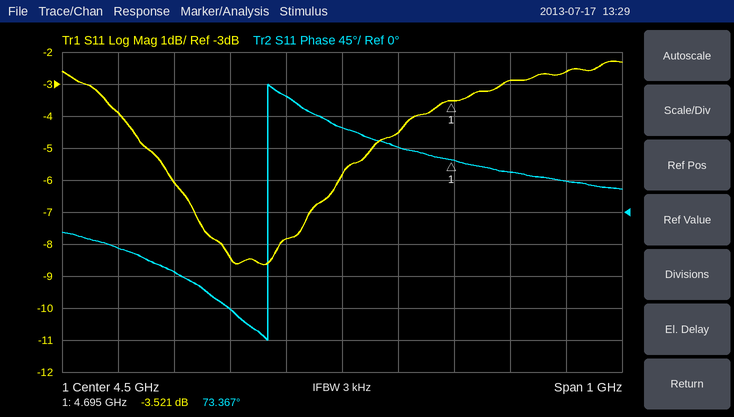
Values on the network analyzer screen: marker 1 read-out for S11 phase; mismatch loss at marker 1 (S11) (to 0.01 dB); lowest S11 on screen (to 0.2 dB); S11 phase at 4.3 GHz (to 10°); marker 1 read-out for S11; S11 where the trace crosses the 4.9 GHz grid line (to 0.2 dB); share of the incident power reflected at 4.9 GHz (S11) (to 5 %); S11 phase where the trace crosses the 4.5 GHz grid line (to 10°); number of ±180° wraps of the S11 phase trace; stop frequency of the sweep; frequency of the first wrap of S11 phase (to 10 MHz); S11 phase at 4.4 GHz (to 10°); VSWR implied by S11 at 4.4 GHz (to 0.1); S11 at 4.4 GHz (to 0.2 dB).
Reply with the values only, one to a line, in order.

73.367°
2.55 dB
-8.6 dB
-140°
-3.521 dB
-2.6 dB
55 %
120°
1
5 GHz
4.37 GHz
160°
2.4
-7.8 dB
